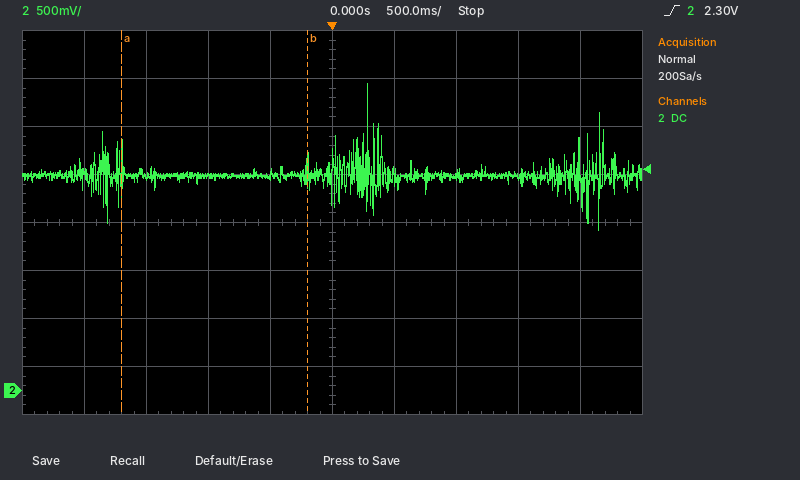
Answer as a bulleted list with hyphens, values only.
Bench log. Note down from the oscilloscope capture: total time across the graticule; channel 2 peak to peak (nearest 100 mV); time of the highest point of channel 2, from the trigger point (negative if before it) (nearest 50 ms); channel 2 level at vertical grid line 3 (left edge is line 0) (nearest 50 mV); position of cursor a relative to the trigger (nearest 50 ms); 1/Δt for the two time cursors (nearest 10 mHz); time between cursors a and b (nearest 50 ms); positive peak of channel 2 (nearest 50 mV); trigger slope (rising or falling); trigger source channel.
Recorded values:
- 5 s
- 1.50 V
- +300 ms
- 2.25 V
- -1.70 s
- 670 mHz
- 1.50 s
- 3.20 V
- rising
- channel 2
